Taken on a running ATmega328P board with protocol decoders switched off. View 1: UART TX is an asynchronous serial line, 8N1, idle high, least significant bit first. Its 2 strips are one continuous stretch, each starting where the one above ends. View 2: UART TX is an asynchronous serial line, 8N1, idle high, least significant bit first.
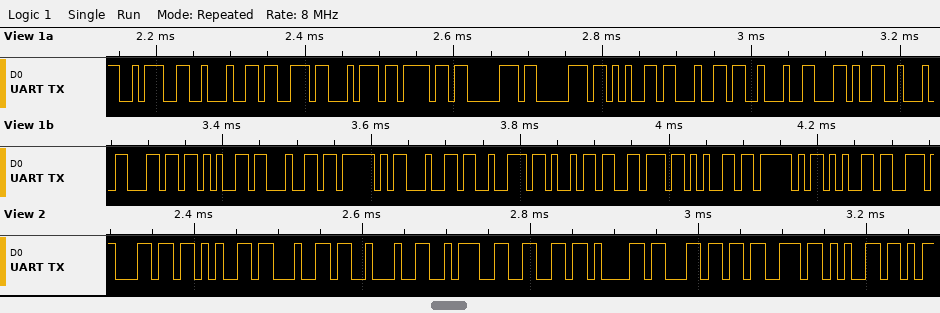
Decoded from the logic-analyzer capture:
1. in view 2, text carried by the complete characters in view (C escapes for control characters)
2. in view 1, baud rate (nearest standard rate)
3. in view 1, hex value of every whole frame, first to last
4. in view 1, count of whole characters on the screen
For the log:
"led\":false"
115200 baud
3A 22 73 74 6F 70 70 65 64 22 2C 22 6C 65 64 5F 64 72 69 76 65 5F 65
23
